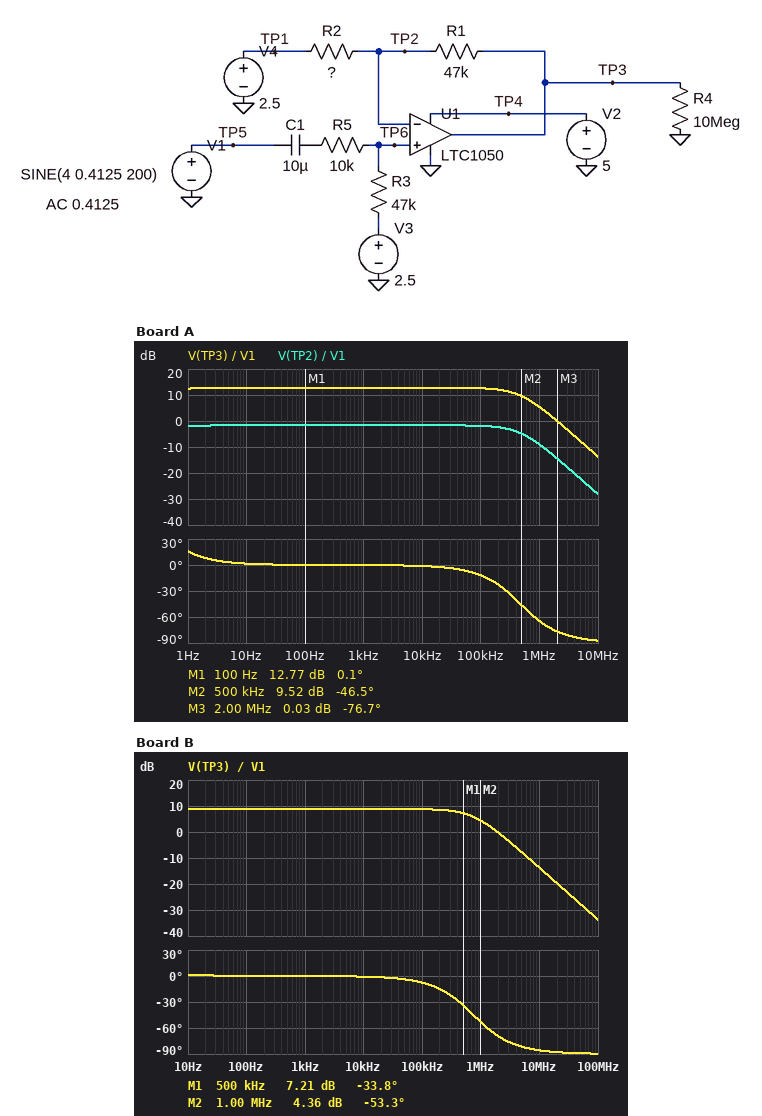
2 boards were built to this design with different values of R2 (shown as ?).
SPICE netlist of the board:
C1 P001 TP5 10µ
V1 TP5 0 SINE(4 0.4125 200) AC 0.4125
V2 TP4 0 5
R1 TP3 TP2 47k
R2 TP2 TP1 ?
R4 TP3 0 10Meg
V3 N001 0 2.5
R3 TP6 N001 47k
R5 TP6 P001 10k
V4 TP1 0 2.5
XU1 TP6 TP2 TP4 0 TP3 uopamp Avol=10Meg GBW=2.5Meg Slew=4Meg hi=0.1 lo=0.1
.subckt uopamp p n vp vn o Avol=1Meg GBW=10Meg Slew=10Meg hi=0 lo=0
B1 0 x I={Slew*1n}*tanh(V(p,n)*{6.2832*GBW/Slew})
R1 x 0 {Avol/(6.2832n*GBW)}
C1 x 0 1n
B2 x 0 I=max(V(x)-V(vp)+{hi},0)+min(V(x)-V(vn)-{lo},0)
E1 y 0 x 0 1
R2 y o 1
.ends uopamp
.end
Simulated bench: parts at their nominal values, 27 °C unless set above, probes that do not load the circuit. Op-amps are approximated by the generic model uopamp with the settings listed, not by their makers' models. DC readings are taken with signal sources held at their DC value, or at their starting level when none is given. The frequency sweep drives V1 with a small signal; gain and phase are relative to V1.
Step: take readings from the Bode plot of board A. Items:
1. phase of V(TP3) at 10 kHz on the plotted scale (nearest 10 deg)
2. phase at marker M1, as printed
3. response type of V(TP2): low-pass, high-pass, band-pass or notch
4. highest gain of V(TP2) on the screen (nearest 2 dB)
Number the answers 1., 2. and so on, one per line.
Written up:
1. 0 deg
2. 0.1 deg
3. low-pass
4. -2 dB
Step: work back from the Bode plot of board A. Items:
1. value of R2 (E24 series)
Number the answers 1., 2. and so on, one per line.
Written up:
1. 11 kΩ
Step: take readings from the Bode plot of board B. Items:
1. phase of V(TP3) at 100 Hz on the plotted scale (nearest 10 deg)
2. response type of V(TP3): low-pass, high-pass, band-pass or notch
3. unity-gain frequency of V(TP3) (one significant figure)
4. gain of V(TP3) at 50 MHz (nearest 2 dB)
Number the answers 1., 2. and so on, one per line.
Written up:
1. 0 deg
2. low-pass
3. 2 MHz
4. -28 dB
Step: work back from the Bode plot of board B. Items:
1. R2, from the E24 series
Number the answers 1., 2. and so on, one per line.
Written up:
1. 20 kΩ
